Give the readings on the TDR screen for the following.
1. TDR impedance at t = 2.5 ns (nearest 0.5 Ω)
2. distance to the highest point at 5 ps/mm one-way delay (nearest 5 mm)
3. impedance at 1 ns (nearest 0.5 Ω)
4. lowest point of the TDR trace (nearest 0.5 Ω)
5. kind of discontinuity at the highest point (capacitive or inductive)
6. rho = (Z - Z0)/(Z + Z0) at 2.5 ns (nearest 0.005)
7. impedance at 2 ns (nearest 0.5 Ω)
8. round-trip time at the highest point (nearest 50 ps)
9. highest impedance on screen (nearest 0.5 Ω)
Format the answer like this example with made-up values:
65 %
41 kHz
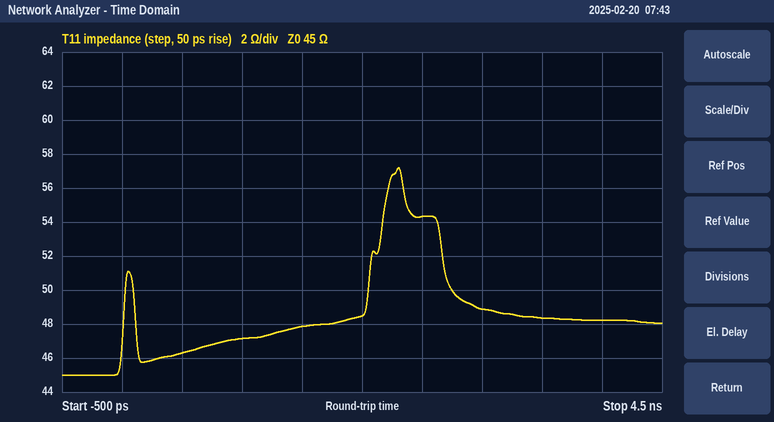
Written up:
54.5 Ω
230 mm
47.0 Ω
45.0 Ω
inductive
+0.095
48.5 Ω
2.30 ns
57.0 Ω
